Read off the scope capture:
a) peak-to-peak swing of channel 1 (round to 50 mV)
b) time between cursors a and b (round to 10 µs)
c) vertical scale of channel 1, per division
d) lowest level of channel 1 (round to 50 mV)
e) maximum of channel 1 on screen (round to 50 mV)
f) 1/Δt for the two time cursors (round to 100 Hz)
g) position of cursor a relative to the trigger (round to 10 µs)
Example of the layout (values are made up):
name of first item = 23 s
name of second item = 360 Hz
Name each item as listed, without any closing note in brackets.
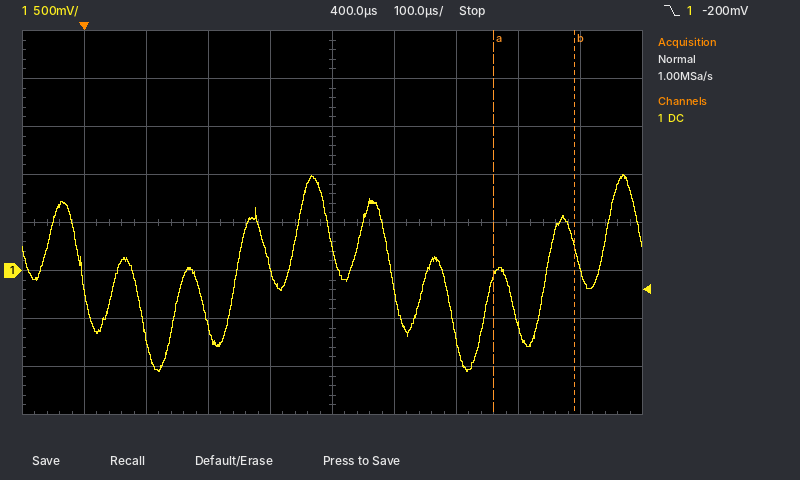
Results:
peak-to-peak swing of channel 1 = 2.05 V
time between cursors a and b = 130 µs
vertical scale of channel 1, per division = 500 mV
lowest level of channel 1 = -1.05 V
maximum of channel 1 on screen = 1.00 V
1/Δt for the two time cursors = 7.7 kHz
position of cursor a relative to the trigger = +660 µs
